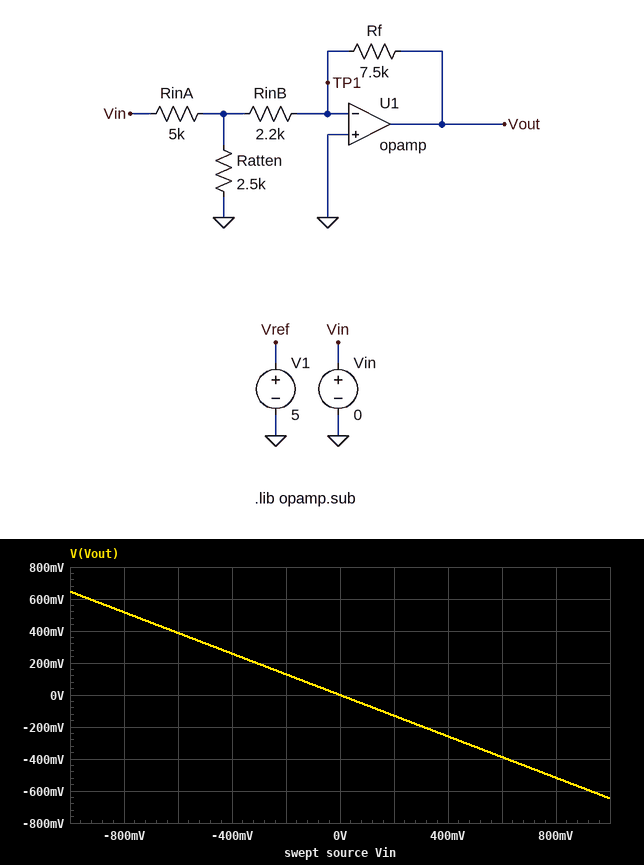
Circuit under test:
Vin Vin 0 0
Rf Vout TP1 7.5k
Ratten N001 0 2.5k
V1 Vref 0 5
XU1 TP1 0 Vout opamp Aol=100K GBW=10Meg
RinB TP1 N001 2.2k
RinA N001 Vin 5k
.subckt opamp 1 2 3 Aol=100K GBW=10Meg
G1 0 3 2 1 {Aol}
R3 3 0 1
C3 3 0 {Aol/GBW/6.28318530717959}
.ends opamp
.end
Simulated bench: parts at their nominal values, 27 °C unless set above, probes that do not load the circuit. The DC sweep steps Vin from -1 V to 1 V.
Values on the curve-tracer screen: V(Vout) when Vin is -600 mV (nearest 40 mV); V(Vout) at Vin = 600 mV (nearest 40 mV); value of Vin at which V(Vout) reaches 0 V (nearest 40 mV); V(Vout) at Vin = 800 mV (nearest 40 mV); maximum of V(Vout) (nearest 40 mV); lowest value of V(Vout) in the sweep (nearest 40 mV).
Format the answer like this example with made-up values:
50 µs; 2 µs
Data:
400 mV; -400 mV; 0 V; -520 mV; 640 mV; -640 mV
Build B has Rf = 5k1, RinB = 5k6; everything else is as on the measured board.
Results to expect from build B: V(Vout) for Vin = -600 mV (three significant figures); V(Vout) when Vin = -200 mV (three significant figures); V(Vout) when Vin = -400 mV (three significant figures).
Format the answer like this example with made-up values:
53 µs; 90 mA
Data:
140 mV; 46.8 mV; 93.6 mV
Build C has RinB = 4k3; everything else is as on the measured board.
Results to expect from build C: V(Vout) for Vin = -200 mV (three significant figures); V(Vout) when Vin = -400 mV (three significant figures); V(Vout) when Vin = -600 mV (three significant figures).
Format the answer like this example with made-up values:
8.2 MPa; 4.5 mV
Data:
83.8 mV; 168 mV; 251 mV
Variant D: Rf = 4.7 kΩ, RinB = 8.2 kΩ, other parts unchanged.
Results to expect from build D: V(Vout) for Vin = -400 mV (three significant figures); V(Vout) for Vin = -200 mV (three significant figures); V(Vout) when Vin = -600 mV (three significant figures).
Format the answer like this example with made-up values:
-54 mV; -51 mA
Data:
63.5 mV; 31.8 mV; 95.3 mV
